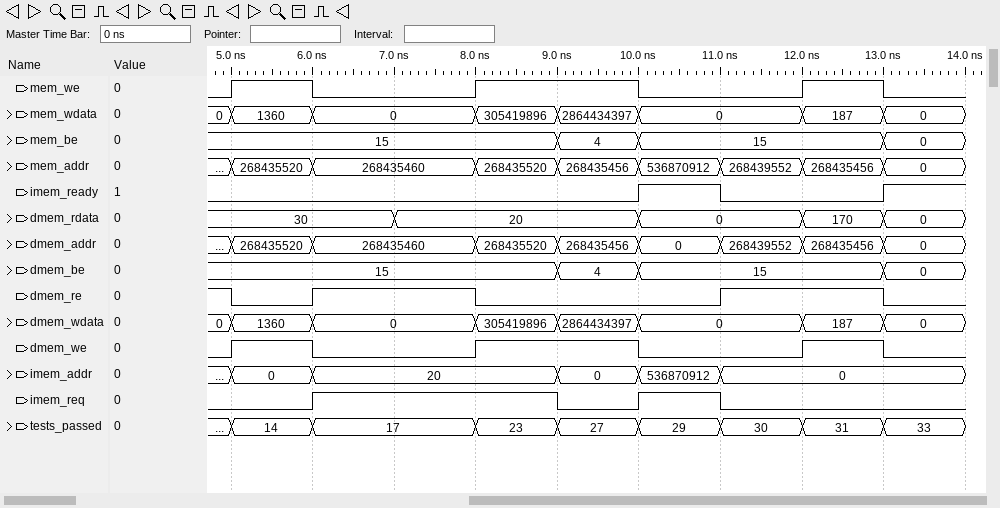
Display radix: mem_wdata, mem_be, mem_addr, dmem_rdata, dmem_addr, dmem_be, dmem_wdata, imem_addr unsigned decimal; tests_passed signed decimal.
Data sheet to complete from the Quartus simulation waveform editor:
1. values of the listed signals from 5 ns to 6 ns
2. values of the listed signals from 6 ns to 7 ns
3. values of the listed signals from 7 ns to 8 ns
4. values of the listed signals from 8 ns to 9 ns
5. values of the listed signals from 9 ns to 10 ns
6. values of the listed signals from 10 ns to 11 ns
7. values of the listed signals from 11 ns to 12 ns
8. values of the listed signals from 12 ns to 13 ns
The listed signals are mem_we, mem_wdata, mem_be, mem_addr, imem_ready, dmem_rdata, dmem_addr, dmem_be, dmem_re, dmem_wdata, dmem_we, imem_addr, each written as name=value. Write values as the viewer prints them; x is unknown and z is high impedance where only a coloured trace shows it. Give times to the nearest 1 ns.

mem_we=1, mem_wdata=1360, mem_be=15, mem_addr=268435520, imem_ready=0, dmem_rdata=30, dmem_addr=268435520, dmem_be=15, dmem_re=0, dmem_wdata=1360, dmem_we=1, imem_addr=0
mem_we=0, mem_wdata=0, mem_be=15, mem_addr=268435460, imem_ready=0, dmem_rdata=30, dmem_addr=268435460, dmem_be=15, dmem_re=1, dmem_wdata=0, dmem_we=0, imem_addr=20
mem_we=0, mem_wdata=0, mem_be=15, mem_addr=268435460, imem_ready=0, dmem_rdata=20, dmem_addr=268435460, dmem_be=15, dmem_re=1, dmem_wdata=0, dmem_we=0, imem_addr=20
mem_we=1, mem_wdata=305419896, mem_be=15, mem_addr=268435520, imem_ready=0, dmem_rdata=20, dmem_addr=268435520, dmem_be=15, dmem_re=0, dmem_wdata=305419896, dmem_we=1, imem_addr=20
mem_we=1, mem_wdata=2864434397, mem_be=4, mem_addr=268435456, imem_ready=0, dmem_rdata=20, dmem_addr=268435456, dmem_be=4, dmem_re=0, dmem_wdata=2864434397, dmem_we=1, imem_addr=0
mem_we=0, mem_wdata=0, mem_be=15, mem_addr=536870912, imem_ready=1, dmem_rdata=0, dmem_addr=0, dmem_be=15, dmem_re=0, dmem_wdata=0, dmem_we=0, imem_addr=536870912
mem_we=0, mem_wdata=0, mem_be=15, mem_addr=268439552, imem_ready=0, dmem_rdata=0, dmem_addr=268439552, dmem_be=15, dmem_re=1, dmem_wdata=0, dmem_we=0, imem_addr=0
mem_we=1, mem_wdata=187, mem_be=15, mem_addr=268435456, imem_ready=0, dmem_rdata=170, dmem_addr=268435456, dmem_be=15, dmem_re=1, dmem_wdata=187, dmem_we=1, imem_addr=0
